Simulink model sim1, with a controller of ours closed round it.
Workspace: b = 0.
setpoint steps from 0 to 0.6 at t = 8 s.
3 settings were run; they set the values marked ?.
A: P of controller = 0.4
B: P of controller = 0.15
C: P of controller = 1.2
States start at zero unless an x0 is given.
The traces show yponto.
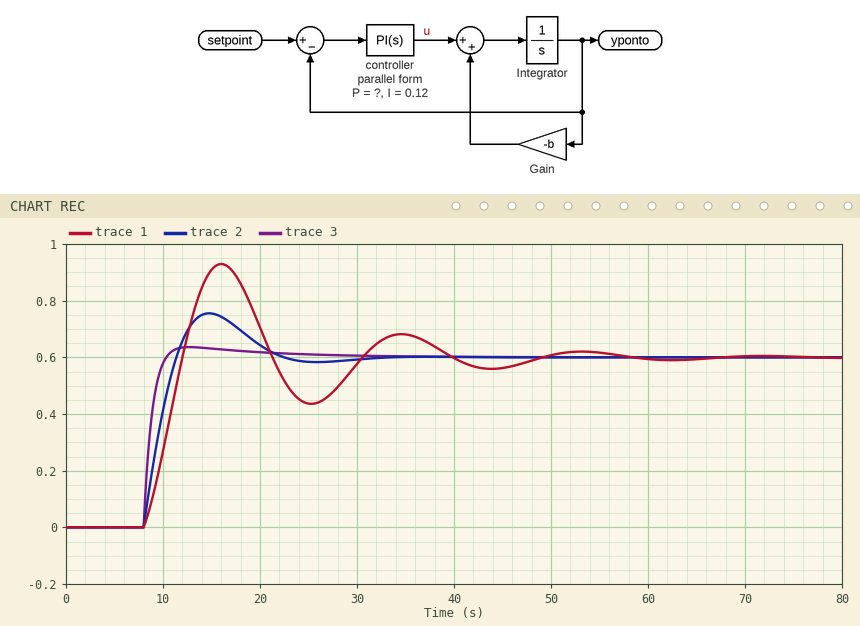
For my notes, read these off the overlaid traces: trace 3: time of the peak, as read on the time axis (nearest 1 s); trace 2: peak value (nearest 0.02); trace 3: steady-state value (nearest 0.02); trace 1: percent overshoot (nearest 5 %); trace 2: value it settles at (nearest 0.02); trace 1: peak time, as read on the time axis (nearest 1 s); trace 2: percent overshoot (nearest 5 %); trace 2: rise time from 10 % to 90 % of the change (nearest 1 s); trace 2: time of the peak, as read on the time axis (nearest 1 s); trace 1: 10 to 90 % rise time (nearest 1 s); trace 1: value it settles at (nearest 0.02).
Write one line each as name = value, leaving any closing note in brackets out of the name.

trace 3: time of the peak, as read on the time axis = 13 s
trace 2: peak value = 0.76
trace 3: steady-state value = 0.60
trace 1: percent overshoot = 55 %
trace 2: value it settles at = 0.60
trace 1: peak time, as read on the time axis = 16 s
trace 2: percent overshoot = 25 %
trace 2: rise time from 10 % to 90 % of the change = 3 s
trace 2: time of the peak, as read on the time axis = 15 s
trace 1: 10 to 90 % rise time = 3 s
trace 1: value it settles at = 0.60
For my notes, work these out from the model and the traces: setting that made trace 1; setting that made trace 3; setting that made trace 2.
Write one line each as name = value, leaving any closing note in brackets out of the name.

setting that made trace 1 = B
setting that made trace 3 = C
setting that made trace 2 = A
